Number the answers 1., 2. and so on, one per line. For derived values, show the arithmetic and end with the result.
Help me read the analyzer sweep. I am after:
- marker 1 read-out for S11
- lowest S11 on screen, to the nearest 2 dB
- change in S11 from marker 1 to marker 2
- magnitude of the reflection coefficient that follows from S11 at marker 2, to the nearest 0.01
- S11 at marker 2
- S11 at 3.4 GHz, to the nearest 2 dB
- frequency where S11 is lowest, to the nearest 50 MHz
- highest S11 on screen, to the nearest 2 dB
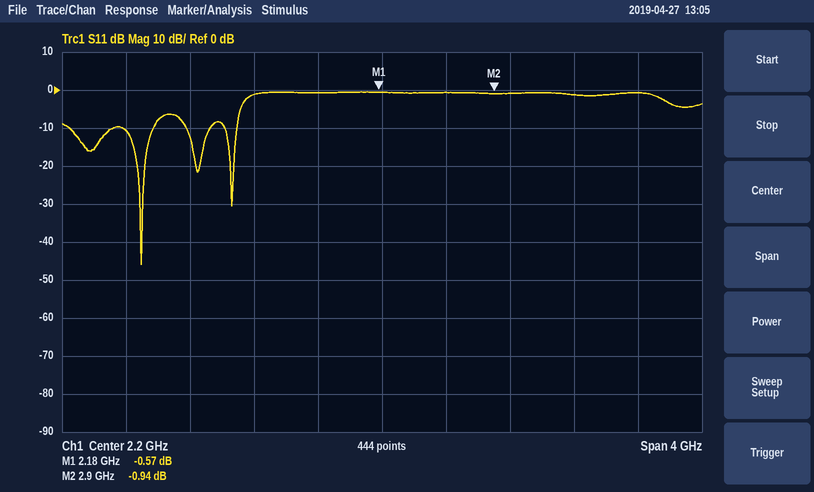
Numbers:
1. -0.57 dB
2. -46 dB
3. -0.94 − (-0.57) = -0.37 dB
4. 10^(-0.94/20) ≈ 0.90
5. -0.94 dB
6. -2 dB
7. 700 MHz
8. 0 dB
